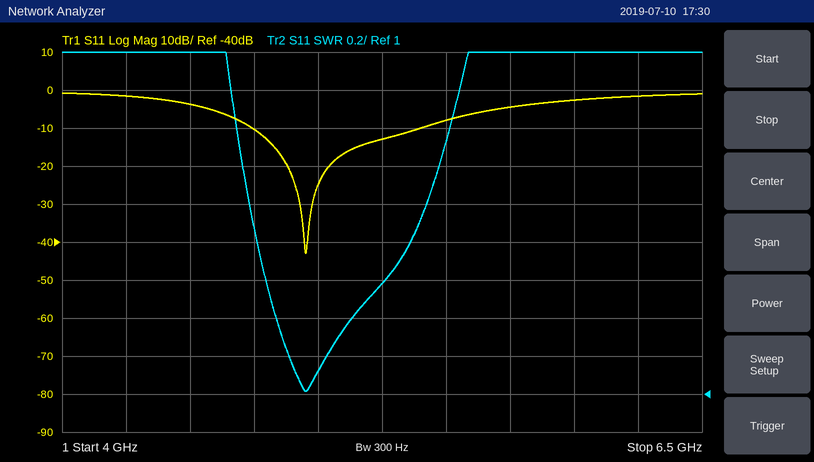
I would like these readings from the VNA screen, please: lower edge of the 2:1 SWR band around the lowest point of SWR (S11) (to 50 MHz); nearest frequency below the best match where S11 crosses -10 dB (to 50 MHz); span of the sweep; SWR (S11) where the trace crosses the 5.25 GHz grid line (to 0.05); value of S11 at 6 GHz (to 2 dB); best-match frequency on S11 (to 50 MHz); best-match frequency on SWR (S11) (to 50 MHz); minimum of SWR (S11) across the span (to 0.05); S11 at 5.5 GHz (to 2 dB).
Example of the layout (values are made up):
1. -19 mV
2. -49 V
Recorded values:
1. 4.75 GHz
2. 4.75 GHz
3. 2.5 GHz
4. 1.60
5. -2 dB
6. 4.95 GHz
7. 4.95 GHz
8. 1.00
9. -8 dB
